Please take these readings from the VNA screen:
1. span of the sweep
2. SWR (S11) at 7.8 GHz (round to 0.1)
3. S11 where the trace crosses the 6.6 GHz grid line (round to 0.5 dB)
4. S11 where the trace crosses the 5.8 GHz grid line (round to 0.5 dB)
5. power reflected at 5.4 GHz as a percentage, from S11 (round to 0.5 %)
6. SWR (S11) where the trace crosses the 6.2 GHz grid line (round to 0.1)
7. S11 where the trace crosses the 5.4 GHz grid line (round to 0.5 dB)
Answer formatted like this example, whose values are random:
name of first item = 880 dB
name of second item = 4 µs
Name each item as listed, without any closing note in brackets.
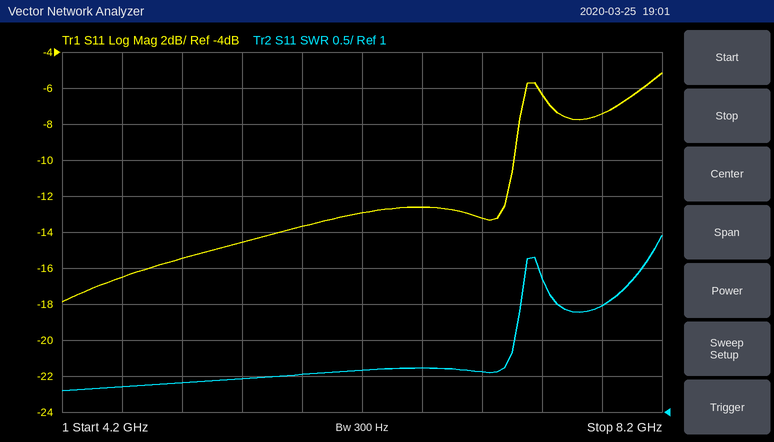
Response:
span of the sweep = 4 GHz
SWR (S11) at 7.8 GHz = 2.5
S11 where the trace crosses the 6.6 GHz grid line = -12.5 dB
S11 where the trace crosses the 5.8 GHz grid line = -13.5 dB
power reflected at 5.4 GHz as a percentage, from S11 = 3.5 %
SWR (S11) where the trace crosses the 6.2 GHz grid line = 1.6
S11 where the trace crosses the 5.4 GHz grid line = -14.5 dB
